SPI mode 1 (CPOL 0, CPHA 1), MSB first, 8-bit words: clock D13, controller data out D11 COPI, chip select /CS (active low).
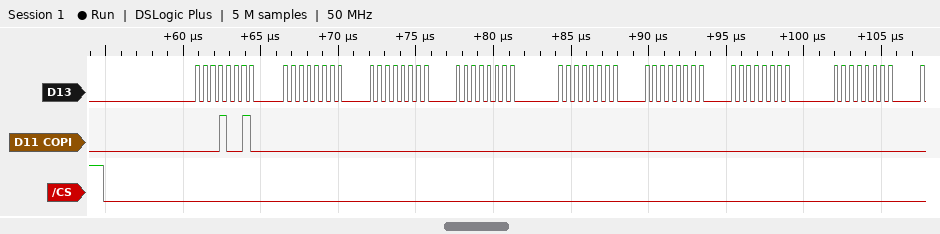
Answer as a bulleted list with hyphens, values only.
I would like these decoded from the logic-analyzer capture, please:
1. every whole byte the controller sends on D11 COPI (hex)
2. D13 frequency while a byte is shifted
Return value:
- 12 00 00 00 00 00 00 00
- 2 MHz
